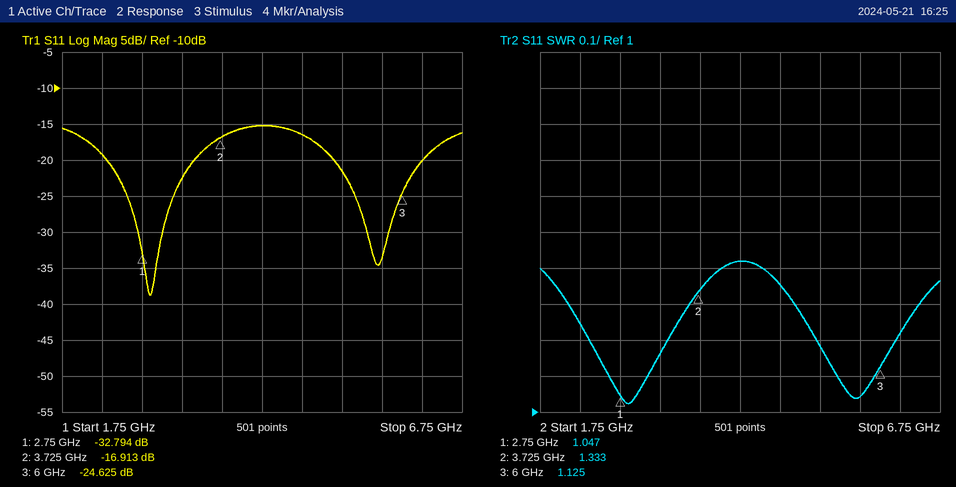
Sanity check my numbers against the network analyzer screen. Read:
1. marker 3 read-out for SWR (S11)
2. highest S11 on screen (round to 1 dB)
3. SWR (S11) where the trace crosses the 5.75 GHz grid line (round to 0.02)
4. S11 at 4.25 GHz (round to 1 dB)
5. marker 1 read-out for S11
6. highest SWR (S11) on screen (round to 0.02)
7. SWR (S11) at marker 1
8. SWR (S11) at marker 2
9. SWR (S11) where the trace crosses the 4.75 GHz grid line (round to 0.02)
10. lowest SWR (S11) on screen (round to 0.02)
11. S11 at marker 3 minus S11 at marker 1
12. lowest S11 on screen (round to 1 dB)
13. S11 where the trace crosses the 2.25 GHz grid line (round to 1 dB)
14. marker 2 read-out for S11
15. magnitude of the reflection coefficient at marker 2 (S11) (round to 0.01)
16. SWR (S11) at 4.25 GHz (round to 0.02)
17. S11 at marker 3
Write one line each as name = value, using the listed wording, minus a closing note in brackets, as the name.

marker 3 read-out for SWR = 1.125
highest S11 on screen = -15 dB
SWR (S11) where the trace crosses the 5.75 GHz grid line = 1.04
S11 at 4.25 GHz = -15 dB
marker 1 read-out for S11 = -32.794 dB
highest SWR (S11) on screen = 1.42
SWR (S11) at marker 1 = 1.047
SWR (S11) at marker 2 = 1.333
SWR (S11) where the trace crosses the 4.75 GHz grid line = 1.36
lowest SWR (S11) on screen = 1.02
S11 at marker 3 minus S11 at marker 1 = 8.169 dB
lowest S11 on screen = -39 dB
S11 where the trace crosses the 2.25 GHz grid line = -19 dB
marker 2 read-out for S11 = -16.913 dB
magnitude of the reflection coefficient at marker 2 (S11) = 0.14
SWR (S11) at 4.25 GHz = 1.42
S11 at marker 3 = -24.625 dB
